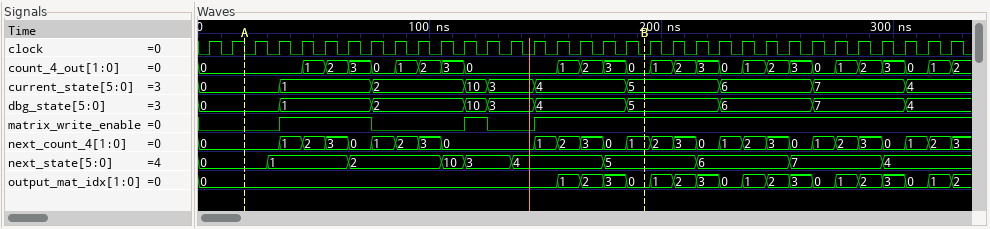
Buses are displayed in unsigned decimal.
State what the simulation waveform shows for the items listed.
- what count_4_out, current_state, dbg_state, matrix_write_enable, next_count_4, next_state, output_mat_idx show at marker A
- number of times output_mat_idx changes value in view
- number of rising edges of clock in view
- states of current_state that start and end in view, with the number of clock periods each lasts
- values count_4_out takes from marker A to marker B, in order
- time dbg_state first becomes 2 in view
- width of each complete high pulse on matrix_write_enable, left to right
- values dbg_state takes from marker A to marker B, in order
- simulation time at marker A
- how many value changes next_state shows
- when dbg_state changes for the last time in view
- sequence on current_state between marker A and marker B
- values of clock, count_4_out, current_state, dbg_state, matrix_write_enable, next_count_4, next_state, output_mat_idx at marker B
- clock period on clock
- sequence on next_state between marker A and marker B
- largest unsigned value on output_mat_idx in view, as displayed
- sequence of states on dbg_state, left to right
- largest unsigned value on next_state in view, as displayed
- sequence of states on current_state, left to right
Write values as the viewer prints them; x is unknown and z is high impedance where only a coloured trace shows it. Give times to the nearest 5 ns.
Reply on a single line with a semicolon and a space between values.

count_4_out=0, current_state=0, dbg_state=0, matrix_write_enable=0, next_count_4=0, next_state=0, output_mat_idx=0; 18; 33; 1: 4, 2: 4, 10: 1, 3: 2, 4: 4, 5: 4, 6: 4, 7: 4; 0, 1, 2, 3, 0, 1, 2, 3, 0, 1, 2, 3, 0; 75 ns; 40 ns, 10 ns; 0, 1, 2, 10, 3, 4, 5; 20 ns; 9; 305 ns; 0, 1, 2, 10, 3, 4, 5; clock=0, count_4_out=0, current_state=5, dbg_state=5, matrix_write_enable=1, next_count_4=1, next_state=5, output_mat_idx=0; 10 ns; 0, 1, 2, 10, 3, 4, 5; 3; 0, 1, 2, 10, 3, 4, 5, 6, 7, 4; 10; 0, 1, 2, 10, 3, 4, 5, 6, 7, 4
